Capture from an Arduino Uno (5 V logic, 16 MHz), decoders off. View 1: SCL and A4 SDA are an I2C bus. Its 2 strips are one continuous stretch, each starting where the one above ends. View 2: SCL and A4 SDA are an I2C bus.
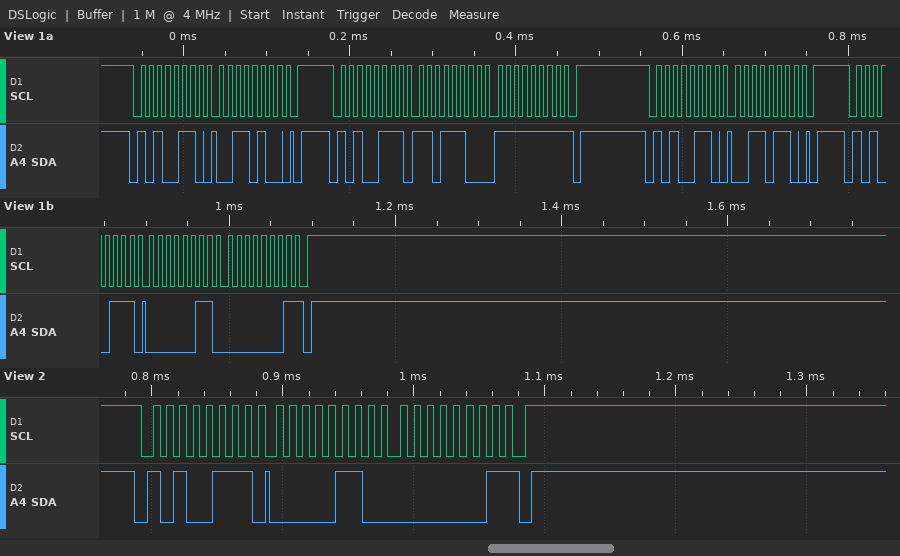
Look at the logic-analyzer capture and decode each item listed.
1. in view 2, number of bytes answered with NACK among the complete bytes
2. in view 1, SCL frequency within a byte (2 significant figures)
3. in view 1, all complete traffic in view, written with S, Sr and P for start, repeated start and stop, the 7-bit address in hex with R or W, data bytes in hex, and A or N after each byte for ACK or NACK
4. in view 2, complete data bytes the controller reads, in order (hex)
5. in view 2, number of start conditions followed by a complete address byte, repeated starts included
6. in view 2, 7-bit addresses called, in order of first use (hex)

1
100 kHz
S 53W A 34 A P S 53R A DC A FF N P S 53W A 36 A P S 53R A 03 A 01 N P
06 01
1
0x53
